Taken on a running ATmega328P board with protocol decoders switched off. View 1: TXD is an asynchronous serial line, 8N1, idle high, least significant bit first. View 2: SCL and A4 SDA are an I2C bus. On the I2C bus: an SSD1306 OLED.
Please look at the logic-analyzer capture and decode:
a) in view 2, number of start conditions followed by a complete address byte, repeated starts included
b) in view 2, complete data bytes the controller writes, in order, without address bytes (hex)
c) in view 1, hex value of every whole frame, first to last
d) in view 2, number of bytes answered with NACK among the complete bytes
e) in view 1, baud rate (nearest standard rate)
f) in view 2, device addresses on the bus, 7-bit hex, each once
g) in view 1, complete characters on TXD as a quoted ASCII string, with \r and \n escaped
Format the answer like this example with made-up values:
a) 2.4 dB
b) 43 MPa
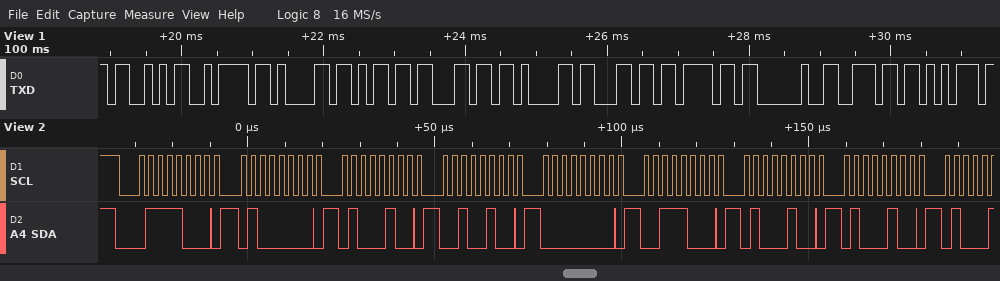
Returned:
a) 1
b) 40 44 24 00 38 44 44
c) 0x53 0x7A 0x61 0x6D 0x6C 0x61 0x6C 0x6F 0x20 0x6E 0x75
d) 0
e) 9600 baud
f) 0x3C
g) "Szamlalo nu"
